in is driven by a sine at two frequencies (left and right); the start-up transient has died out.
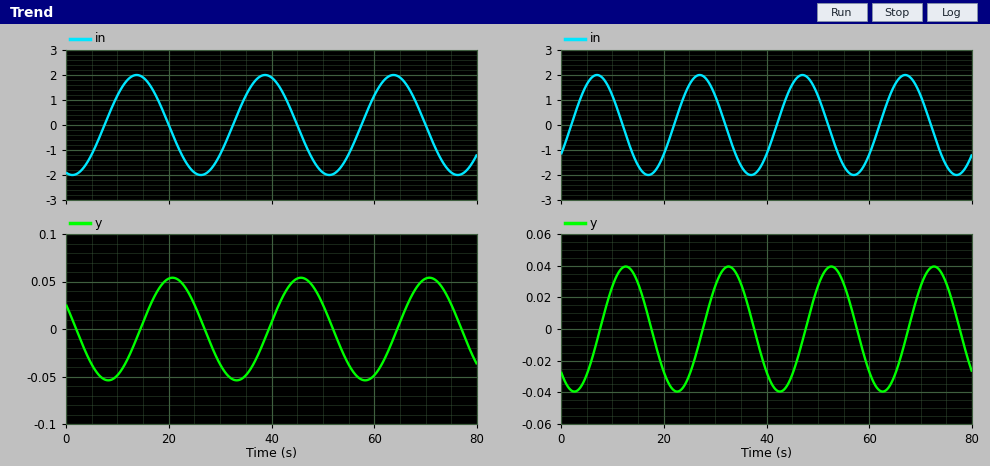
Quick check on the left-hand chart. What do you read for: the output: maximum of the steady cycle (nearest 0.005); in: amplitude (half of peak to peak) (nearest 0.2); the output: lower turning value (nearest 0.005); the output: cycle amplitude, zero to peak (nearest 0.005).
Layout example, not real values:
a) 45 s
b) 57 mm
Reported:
a) 0.055
b) 2.0
c) -0.055
d) 0.055
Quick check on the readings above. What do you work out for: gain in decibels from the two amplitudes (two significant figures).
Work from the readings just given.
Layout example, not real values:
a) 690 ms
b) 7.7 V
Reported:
a) -31 dB
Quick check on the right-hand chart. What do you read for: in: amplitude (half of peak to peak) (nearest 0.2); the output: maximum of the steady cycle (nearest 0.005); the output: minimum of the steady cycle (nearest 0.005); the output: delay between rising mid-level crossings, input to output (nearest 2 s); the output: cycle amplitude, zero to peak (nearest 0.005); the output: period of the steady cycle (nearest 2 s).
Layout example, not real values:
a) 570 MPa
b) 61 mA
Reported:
a) 2.0
b) 0.040
c) -0.040
d) 6 s
e) 0.040
f) 20 s
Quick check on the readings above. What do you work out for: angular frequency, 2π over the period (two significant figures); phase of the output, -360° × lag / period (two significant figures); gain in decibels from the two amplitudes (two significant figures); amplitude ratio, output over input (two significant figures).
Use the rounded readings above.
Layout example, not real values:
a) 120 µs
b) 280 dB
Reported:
a) 0.31 rad/s
b) -110°
c) -34 dB
d) 0.020
